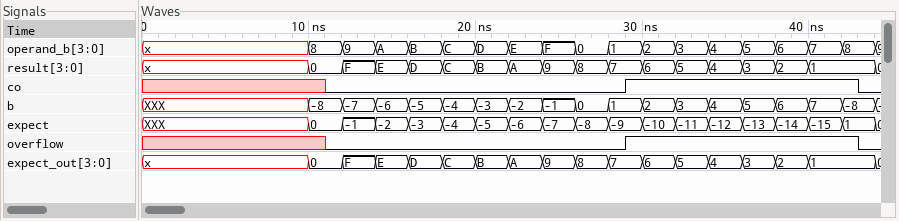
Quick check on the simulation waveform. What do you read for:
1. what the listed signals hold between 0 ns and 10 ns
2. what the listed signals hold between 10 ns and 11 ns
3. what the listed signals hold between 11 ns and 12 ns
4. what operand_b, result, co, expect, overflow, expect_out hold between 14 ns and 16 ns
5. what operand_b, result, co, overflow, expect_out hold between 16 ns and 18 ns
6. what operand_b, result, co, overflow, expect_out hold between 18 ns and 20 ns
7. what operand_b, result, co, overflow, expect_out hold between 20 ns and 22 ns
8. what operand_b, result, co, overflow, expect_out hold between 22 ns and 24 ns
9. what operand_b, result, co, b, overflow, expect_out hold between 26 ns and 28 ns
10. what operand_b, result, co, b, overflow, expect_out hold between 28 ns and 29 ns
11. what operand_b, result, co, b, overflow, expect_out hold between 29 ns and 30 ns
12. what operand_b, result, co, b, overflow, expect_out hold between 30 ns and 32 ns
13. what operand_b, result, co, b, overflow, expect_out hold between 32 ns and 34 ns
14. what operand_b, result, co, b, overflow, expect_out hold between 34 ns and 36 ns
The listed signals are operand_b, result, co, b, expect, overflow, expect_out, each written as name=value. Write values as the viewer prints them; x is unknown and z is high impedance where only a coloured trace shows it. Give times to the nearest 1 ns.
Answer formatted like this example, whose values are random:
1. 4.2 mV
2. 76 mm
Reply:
1. operand_b=x, result=x, co=x, b=XXX, expect=XXX, overflow=x, expect_out=x
2. operand_b=8, result=0, co=x, b=-8, expect=0, overflow=x, expect_out=0
3. operand_b=8, result=0, co=0, b=-8, expect=0, overflow=0, expect_out=0
4. operand_b=A, result=E, co=0, expect=-2, overflow=0, expect_out=E
5. operand_b=B, result=D, co=0, overflow=0, expect_out=D
6. operand_b=C, result=C, co=0, overflow=0, expect_out=C
7. operand_b=D, result=B, co=0, overflow=0, expect_out=B
8. operand_b=E, result=A, co=0, overflow=0, expect_out=A
9. operand_b=0, result=8, co=0, b=0, overflow=0, expect_out=8
10. operand_b=1, result=7, co=0, b=1, overflow=0, expect_out=7
11. operand_b=1, result=7, co=1, b=1, overflow=1, expect_out=7
12. operand_b=2, result=6, co=1, b=2, overflow=1, expect_out=6
13. operand_b=3, result=5, co=1, b=3, overflow=1, expect_out=5
14. operand_b=4, result=4, co=1, b=4, overflow=1, expect_out=4
